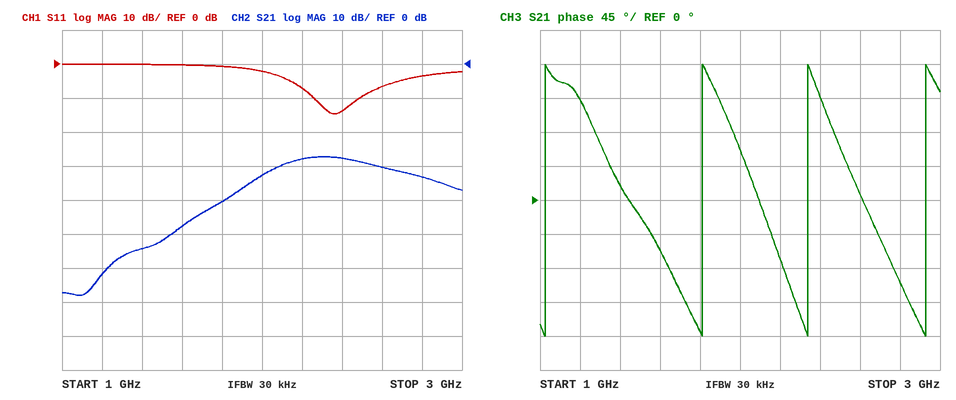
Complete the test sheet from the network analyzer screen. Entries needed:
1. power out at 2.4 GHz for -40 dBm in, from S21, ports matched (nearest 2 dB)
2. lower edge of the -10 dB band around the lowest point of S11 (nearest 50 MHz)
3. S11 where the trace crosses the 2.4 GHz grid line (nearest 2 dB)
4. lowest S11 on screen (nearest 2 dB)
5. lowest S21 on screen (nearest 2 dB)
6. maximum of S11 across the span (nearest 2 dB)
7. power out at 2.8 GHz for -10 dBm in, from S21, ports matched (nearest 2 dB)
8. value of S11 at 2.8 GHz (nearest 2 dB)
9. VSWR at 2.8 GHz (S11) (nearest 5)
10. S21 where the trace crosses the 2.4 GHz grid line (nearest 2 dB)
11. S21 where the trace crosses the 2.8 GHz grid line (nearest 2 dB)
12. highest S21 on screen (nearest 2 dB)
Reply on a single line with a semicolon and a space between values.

-68 dBm; 2.25 GHz; -14 dB; -14 dB; -68 dB; 0 dB; -44 dBm; -4 dB; 5; -28 dB; -34 dB; -28 dB
